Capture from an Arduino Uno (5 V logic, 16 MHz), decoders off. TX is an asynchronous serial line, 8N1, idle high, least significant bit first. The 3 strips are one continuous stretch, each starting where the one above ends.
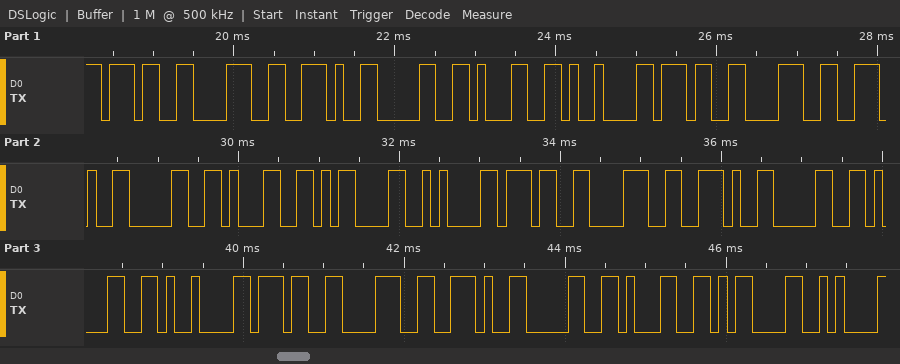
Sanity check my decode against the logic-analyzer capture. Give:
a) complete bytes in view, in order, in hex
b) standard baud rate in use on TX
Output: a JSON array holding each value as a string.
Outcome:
["37 38 2E 30 31 09 37 38 2E 30 31 0D 0A 37 38 2E 30 31 09 37 38 2E 30 31 0D 0A", "9600 baud"]
